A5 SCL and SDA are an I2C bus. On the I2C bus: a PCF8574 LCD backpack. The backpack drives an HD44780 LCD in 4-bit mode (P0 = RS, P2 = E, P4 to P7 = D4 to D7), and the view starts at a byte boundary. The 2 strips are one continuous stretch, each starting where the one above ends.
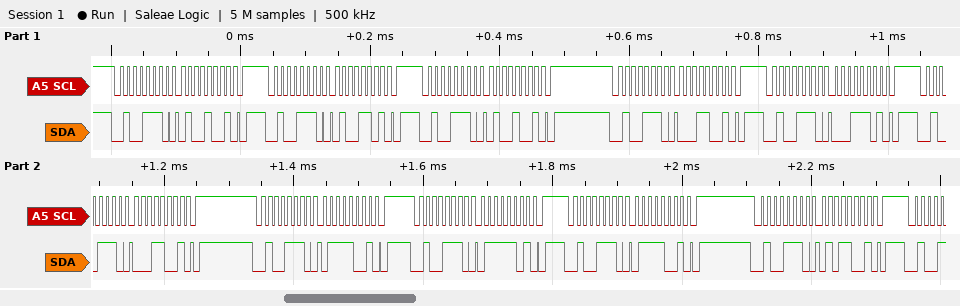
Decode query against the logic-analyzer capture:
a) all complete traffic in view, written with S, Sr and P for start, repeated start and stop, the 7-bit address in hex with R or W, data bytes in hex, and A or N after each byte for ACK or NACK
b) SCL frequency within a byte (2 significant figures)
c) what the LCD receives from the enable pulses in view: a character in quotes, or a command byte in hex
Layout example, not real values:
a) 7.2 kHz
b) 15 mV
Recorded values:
a) S 27W A 49 A P S 27W A 4D A P S 27W A 49 A P S 27W A 19 A P S 27W A 1D A P S 27W A 19 A P S 27W A 79 A P S 27W A 7D A P S 27W A 79 A P S 27W A 59 A P
b) 100 kHz
c) 'A'
